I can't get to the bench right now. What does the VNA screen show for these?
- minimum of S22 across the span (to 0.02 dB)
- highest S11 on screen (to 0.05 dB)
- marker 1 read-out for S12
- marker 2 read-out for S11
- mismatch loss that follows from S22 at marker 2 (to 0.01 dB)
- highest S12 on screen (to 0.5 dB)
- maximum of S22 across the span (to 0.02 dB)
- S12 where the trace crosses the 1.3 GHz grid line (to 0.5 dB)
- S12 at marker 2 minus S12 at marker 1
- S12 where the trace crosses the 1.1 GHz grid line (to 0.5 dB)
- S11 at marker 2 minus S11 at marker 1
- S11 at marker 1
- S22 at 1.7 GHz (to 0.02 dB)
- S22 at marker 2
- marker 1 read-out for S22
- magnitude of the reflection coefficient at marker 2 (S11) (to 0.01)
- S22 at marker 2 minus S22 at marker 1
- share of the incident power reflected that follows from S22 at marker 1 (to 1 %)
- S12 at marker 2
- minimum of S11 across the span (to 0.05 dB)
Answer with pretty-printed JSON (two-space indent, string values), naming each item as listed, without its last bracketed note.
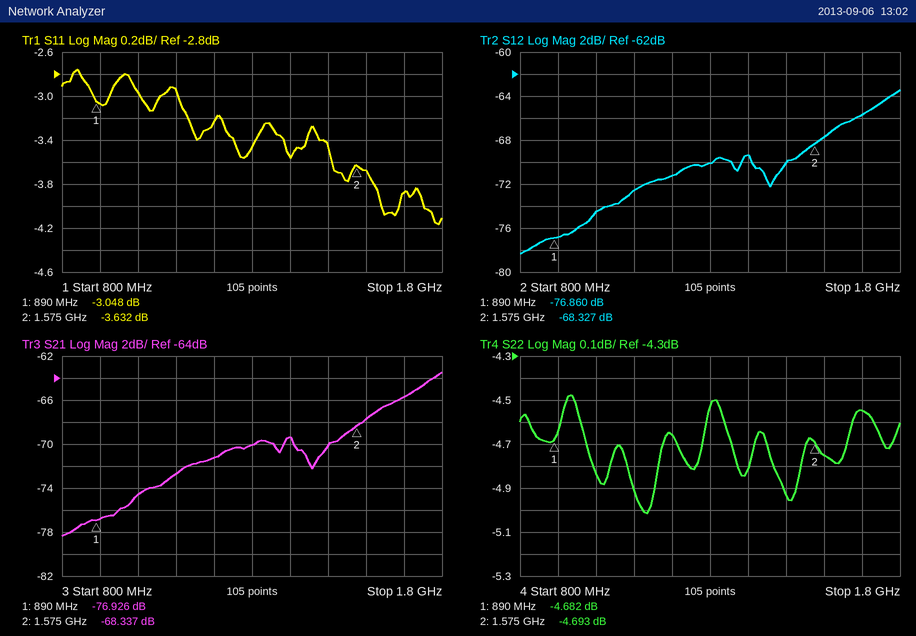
{
  "minimum of S22 across the span": "-5.02 dB",
  "highest S11 on screen": "-2.75 dB",
  "marker 1 read-out for S12": "-76.860 dB",
  "marker 2 read-out for S11": "-3.632 dB",
  "mismatch loss that follows from S22 at marker 2": "1.80 dB",
  "highest S12 on screen": "-63.5 dB",
  "maximum of S22 across the span": "-4.48 dB",
  "S12 where the trace crosses the 1.3 GHz grid line": "-70.0 dB",
  "S12 at marker 2 minus S12 at marker 1": "8.533 dB",
  "S12 where the trace crosses the 1.1 GHz grid line": "-72.5 dB",
  "S11 at marker 2 minus S11 at marker 1": "-0.584 dB",
  "S11 at marker 1": "-3.048 dB",
  "S22 at 1.7 GHz": "-4.54 dB",
  "S22 at marker 2": "-4.693 dB",
  "marker 1 read-out for S22": "-4.682 dB",
  "magnitude of the reflection coefficient at marker 2 (S11)": "0.66",
  "S22 at marker 2 minus S22 at marker 1": "-0.011 dB",
  "share of the incident power reflected that follows from S22 at marker 1": "34 %",
  "S12 at marker 2": "-68.327 dB",
  "minimum of S11 across the span": "-4.15 dB"
}
